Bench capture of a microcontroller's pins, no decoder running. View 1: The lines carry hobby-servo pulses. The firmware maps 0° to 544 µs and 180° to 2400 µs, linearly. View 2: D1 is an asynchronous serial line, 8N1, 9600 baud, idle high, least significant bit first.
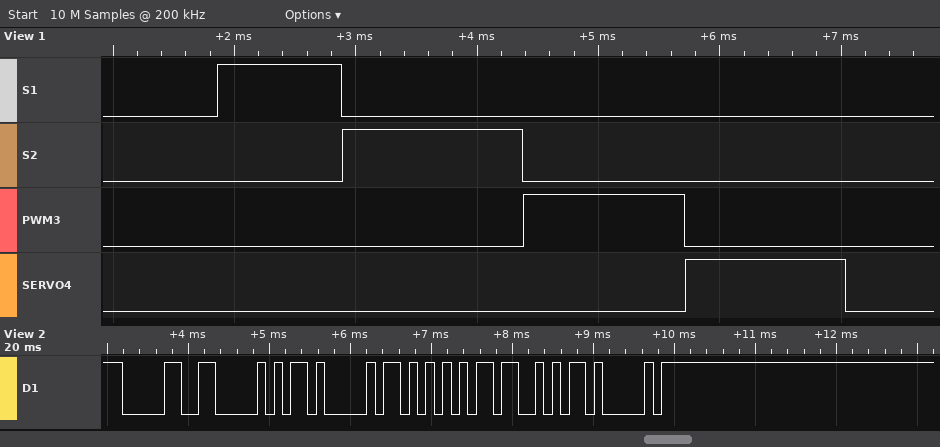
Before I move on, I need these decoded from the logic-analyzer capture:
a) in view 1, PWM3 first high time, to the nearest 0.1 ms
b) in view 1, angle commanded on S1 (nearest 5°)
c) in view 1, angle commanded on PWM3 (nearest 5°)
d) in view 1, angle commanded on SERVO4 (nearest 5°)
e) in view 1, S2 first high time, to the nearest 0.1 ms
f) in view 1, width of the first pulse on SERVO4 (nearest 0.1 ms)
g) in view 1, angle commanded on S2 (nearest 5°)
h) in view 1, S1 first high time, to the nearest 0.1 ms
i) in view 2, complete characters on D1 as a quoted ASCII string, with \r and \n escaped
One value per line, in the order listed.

1.3 ms
45°
75°
75°
1.5 ms
1.3 ms
90°
1.0 ms
"0PAUSA"
